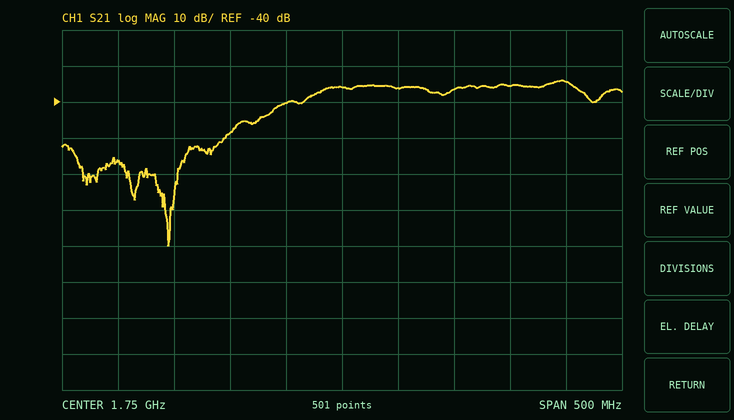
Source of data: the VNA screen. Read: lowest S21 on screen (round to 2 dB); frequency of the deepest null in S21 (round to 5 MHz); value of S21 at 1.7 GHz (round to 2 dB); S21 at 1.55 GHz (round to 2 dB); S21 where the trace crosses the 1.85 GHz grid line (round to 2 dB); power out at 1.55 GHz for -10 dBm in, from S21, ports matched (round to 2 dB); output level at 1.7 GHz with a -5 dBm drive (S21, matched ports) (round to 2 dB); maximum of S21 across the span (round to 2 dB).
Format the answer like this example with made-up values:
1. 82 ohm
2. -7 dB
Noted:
1. -80 dB
2. 1.595 GHz
3. -40 dB
4. -56 dB
5. -36 dB
6. -66 dBm
7. -46 dBm
8. -34 dB
